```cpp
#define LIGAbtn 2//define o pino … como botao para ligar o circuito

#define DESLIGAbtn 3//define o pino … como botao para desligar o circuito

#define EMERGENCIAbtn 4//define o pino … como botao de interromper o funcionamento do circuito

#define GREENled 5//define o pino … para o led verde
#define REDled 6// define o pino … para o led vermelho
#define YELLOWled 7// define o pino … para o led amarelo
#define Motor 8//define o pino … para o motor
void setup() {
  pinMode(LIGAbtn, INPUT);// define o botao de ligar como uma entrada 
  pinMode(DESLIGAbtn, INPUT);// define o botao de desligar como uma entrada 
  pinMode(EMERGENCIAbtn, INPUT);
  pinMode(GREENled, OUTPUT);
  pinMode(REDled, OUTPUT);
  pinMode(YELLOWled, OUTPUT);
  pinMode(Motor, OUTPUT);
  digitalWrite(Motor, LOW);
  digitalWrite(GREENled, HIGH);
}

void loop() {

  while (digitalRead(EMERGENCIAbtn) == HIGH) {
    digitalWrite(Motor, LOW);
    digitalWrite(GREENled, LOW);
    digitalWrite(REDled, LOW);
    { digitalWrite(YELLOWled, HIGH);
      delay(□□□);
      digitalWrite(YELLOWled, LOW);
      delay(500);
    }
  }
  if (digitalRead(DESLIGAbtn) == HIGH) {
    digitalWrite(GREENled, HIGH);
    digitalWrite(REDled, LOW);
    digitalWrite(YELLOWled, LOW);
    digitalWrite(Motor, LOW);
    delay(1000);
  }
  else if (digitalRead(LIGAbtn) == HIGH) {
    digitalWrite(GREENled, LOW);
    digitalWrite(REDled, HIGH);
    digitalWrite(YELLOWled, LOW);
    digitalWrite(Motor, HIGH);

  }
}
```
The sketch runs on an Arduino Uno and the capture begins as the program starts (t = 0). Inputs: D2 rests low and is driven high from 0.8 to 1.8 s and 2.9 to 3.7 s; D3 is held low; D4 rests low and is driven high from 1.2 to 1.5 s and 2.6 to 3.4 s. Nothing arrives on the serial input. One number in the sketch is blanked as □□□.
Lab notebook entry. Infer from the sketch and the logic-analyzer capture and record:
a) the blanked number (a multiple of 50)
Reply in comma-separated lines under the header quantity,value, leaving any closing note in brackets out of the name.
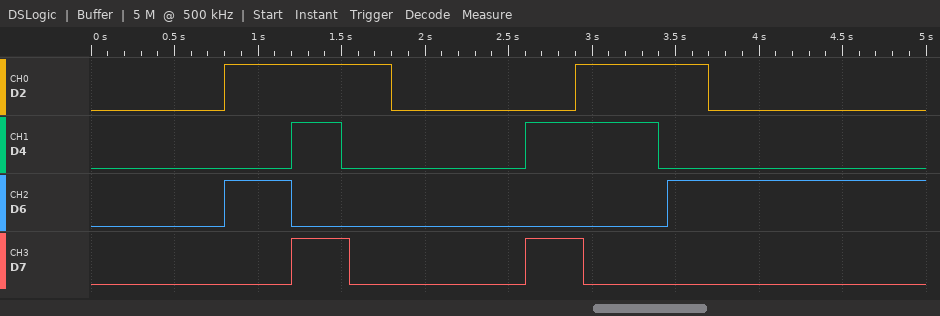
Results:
quantity,value
the blanked number,350
